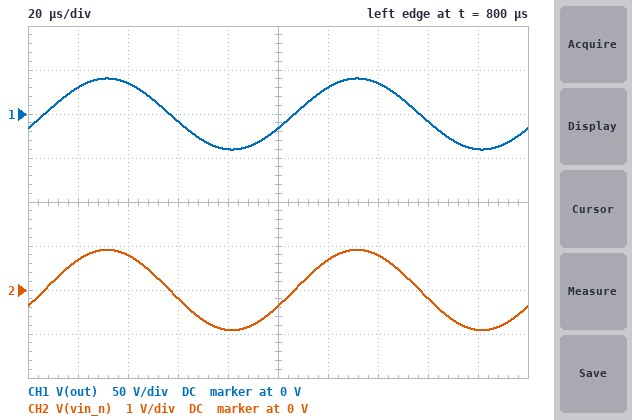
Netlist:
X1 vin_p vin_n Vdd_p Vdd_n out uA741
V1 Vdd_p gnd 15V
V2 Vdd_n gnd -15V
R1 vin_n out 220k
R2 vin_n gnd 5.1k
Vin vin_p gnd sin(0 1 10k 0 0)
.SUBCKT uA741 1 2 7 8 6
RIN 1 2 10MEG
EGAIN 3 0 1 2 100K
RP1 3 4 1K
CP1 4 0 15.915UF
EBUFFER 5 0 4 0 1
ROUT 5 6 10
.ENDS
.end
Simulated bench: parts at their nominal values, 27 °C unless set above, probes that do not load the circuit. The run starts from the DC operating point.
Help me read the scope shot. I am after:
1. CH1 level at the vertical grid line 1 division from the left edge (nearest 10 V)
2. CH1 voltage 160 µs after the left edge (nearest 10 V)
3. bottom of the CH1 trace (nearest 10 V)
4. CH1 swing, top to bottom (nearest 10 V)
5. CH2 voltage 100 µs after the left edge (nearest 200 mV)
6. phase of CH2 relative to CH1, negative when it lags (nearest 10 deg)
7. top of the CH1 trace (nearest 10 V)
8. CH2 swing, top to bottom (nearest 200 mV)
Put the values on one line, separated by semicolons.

30 V; -10 V; -40 V; 80 V; -400 mV; 0 deg; 40 V; 1.8 V
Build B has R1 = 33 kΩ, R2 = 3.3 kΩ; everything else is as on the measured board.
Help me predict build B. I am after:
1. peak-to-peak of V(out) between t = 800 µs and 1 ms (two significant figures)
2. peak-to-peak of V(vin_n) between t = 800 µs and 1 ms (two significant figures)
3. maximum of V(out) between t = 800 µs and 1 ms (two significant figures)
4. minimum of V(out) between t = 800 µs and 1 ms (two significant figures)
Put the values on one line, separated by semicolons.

22 V; 2.0 V; 11 V; -11 V
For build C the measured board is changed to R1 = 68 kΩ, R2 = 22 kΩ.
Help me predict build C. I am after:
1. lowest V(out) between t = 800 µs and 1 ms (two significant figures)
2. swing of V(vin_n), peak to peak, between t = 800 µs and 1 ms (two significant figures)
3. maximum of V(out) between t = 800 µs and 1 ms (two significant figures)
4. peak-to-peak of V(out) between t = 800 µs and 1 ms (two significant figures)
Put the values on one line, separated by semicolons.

-4.1 V; 2.0 V; 4.1 V; 8.2 V
